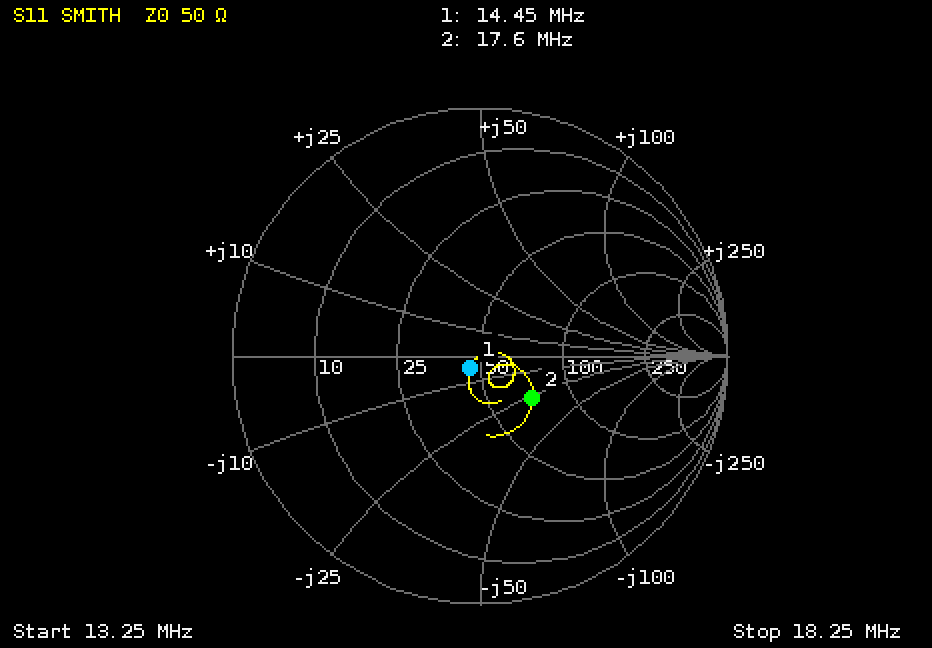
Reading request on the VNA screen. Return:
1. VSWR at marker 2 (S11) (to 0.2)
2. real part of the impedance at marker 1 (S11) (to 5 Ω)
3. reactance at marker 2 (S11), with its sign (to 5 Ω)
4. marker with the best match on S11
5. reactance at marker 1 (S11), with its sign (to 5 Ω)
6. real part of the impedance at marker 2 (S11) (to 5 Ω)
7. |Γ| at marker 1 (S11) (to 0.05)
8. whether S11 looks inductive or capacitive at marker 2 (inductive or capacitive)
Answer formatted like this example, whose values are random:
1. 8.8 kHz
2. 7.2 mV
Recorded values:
1. 1.8
2. 45 Ω
3. -25 Ω
4. marker 1
5. -5 Ω
6. 70 Ω
7. 0.05
8. capacitive
